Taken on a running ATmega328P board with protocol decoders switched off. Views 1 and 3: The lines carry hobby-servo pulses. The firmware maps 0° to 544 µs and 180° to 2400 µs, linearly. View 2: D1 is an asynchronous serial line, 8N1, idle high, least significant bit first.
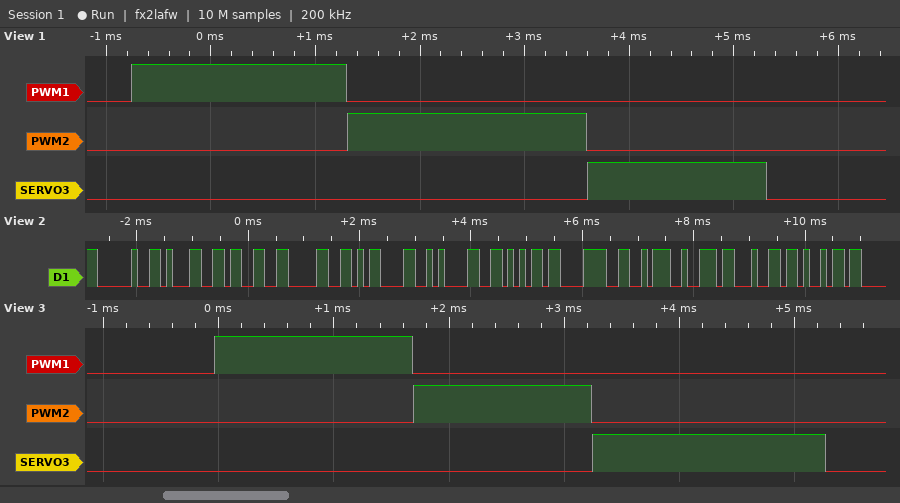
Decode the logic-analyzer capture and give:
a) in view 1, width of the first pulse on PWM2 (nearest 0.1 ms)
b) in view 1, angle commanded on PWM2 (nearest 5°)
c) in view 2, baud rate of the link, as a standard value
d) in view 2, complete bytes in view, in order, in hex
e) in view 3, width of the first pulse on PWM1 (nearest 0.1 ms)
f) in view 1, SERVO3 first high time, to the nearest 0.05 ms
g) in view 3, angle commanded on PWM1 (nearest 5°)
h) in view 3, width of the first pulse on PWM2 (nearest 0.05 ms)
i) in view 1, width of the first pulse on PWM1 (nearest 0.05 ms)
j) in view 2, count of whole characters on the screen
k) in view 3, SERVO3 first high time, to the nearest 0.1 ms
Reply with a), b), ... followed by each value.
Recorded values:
a) 2.3 ms
b) 170°
c) 9600 baud
d) 20 31 33 30 0D 0A 56 C3 A6 72 64 69
e) 1.7 ms
f) 1.70 ms
g) 115°
h) 1.55 ms
i) 2.05 ms
j) 12
k) 2.0 ms
